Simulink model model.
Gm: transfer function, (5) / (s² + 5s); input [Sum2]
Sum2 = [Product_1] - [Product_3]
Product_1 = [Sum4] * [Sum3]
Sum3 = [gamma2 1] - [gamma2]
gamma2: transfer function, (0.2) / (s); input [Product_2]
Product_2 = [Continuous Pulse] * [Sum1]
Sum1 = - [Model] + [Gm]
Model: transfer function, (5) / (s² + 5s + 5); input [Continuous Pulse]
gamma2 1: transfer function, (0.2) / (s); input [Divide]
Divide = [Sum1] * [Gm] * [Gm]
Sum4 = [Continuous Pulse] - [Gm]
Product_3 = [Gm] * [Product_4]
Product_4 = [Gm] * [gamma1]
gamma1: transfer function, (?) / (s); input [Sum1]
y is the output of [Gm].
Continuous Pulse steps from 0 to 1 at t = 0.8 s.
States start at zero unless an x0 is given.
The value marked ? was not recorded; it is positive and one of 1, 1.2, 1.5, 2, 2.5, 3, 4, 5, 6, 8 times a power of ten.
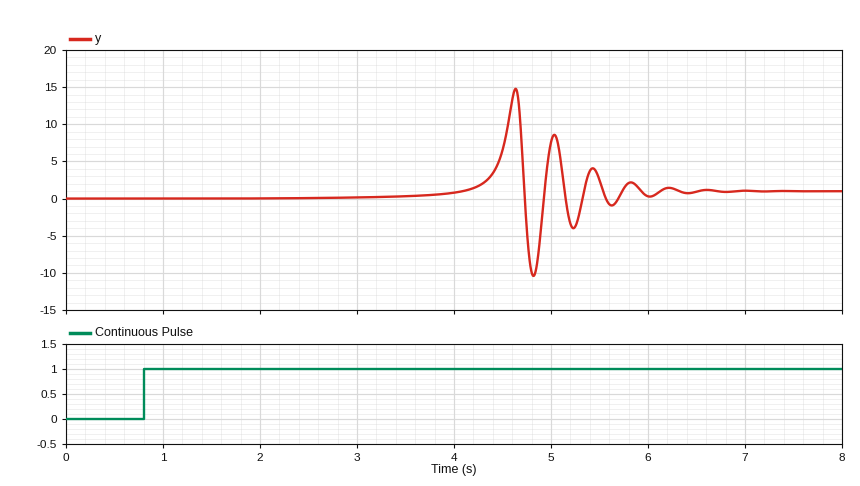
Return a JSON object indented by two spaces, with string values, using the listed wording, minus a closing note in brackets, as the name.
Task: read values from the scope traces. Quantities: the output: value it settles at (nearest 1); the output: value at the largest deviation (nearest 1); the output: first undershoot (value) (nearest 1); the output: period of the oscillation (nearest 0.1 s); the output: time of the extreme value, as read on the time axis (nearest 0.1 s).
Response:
{
  "the output: value it settles at": "1",
  "the output: value at the largest deviation": "15",
  "the output: first undershoot (value)": "-10",
  "the output: period of the oscillation": "0.4 s",
  "the output: time of the extreme value, as read on the time axis": "4.6 s"
}
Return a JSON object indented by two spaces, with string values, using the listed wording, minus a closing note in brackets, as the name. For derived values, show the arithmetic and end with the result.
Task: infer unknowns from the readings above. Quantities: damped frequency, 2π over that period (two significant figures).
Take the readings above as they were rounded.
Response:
{
  "damped frequency, 2π over that period": "2π / 0.4 = 16 rad/s"
}
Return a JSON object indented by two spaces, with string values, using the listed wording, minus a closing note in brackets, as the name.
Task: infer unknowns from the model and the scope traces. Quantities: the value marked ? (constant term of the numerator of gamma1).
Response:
{
  "the value marked ?": "3"
}
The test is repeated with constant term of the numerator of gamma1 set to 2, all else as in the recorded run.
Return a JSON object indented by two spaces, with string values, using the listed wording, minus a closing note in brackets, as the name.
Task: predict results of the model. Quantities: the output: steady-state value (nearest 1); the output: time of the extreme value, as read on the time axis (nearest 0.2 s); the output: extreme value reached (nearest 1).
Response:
{
  "the output: steady-state value": "1",
  "the output: time of the extreme value, as read on the time axis": "5.0 s",
  "the output: extreme value reached": "11"
}
